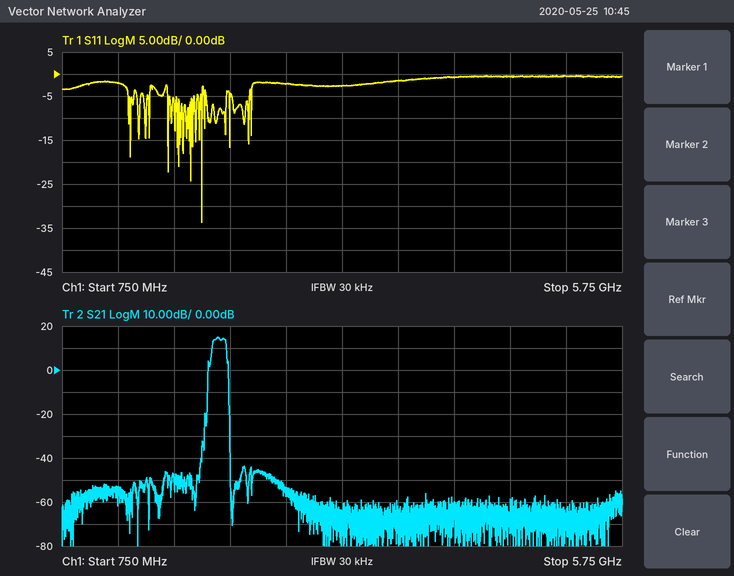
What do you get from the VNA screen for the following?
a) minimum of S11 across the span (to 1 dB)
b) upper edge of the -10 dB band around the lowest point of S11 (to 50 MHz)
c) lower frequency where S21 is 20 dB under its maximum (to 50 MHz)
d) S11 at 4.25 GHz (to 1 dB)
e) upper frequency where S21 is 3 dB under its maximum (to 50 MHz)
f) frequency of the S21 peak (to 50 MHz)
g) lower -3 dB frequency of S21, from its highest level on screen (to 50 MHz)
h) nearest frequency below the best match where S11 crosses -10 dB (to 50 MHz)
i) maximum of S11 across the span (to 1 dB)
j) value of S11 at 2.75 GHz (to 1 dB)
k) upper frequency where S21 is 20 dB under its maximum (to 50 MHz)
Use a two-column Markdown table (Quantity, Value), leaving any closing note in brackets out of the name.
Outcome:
| Quantity | Value |
|---|---|
| minimum of S11 across the span | -34 dB |
| upper edge of the -10 dB band around the lowest point of S11 | 2.00 GHz |
| lower frequency where S21 is 20 dB under its maximum | 2.05 GHz |
| S11 at 4.25 GHz | -1 dB |
| upper frequency where S21 is 3 dB under its maximum | 2.20 GHz |
| frequency of the S21 peak | 2.15 GHz |
| lower -3 dB frequency of S21, from its highest level on screen | 2.10 GHz |
| nearest frequency below the best match where S11 crosses -10 dB | 2.00 GHz |
| maximum of S11 across the span | 0 dB |
| value of S11 at 2.75 GHz | -2 dB |
| upper frequency where S21 is 20 dB under its maximum | 2.25 GHz |
